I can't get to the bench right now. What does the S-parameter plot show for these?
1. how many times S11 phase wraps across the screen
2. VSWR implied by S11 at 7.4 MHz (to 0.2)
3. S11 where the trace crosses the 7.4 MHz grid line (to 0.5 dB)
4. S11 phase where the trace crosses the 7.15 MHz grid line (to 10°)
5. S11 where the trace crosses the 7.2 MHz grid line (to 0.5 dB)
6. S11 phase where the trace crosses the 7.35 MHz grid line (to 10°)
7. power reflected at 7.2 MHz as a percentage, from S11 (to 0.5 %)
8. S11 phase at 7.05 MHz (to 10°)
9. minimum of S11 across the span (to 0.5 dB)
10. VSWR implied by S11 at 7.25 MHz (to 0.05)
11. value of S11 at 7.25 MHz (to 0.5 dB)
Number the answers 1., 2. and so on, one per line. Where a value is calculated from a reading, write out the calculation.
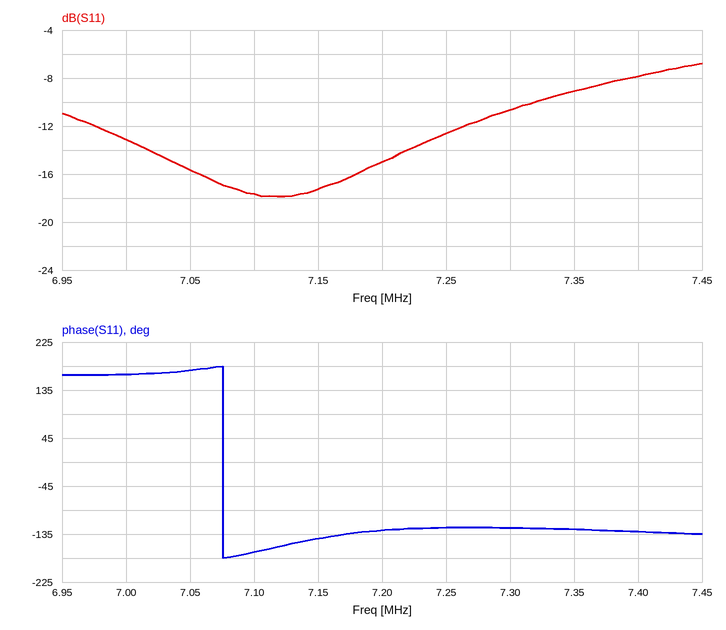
1. 1
2. |Γ| = 10^(-8/20) = 0.3981; VSWR = (1 + 0.3981)/(1 − 0.3981) ≈ 2.32, so 2.4 to the nearest 0.2
3. -8.0 dB
4. -140°
5. -15.0 dB
6. -130°
7. 10^(-15/10) ≈ 3.16 %, so 3.0 % to the nearest 0.5 %
8. 170°
9. -18.0 dB
10. |Γ| = 10^(-12.5/20) = 0.2371; VSWR = (1 + 0.2371)/(1 − 0.2371) ≈ 1.62, so 1.60 to the nearest 0.05
11. -12.5 dB
